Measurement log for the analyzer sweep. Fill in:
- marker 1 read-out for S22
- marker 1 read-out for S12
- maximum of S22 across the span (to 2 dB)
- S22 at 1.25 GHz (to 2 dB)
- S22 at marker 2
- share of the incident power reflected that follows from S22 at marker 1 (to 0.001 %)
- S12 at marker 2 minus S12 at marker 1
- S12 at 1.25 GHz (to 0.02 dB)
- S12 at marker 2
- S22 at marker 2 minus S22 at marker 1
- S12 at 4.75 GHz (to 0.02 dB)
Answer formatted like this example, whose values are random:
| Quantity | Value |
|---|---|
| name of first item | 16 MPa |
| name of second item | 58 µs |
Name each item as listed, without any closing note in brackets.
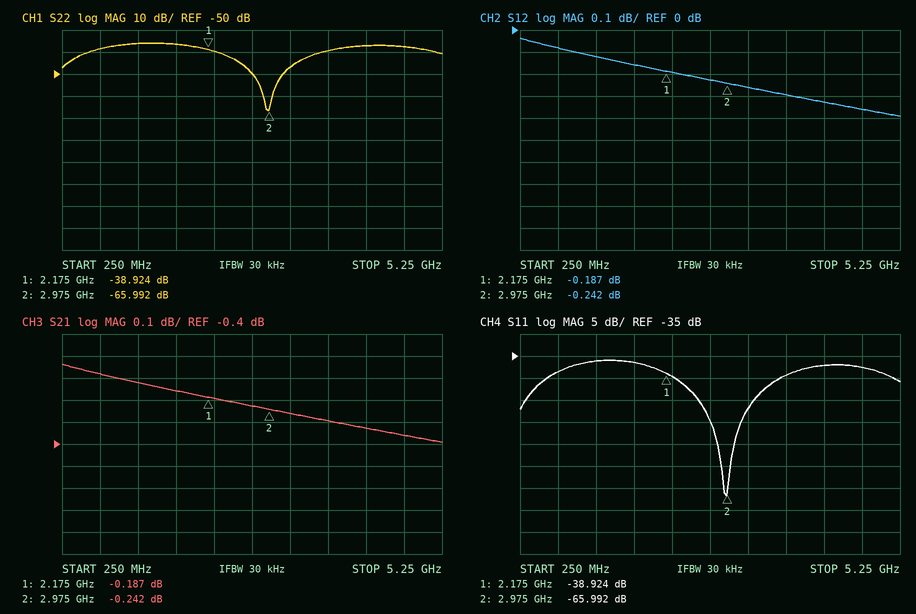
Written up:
| Quantity | Value |
|---|---|
| marker 1 read-out for S22 | -38.924 dB |
| marker 1 read-out for S12 | -0.187 dB |
| maximum of S22 across the span | -36 dB |
| S22 at 1.25 GHz | -36 dB |
| S22 at marker 2 | -65.992 dB |
| share of the incident power reflected that follows from S22 at marker 1 | 0.013 % |
| S12 at marker 2 minus S12 at marker 1 | -0.055 dB |
| S12 at 1.25 GHz | -0.12 dB |
| S12 at marker 2 | -0.242 dB |
| S22 at marker 2 minus S22 at marker 1 | -27.068 dB |
| S12 at 4.75 GHz | -0.36 dB |
